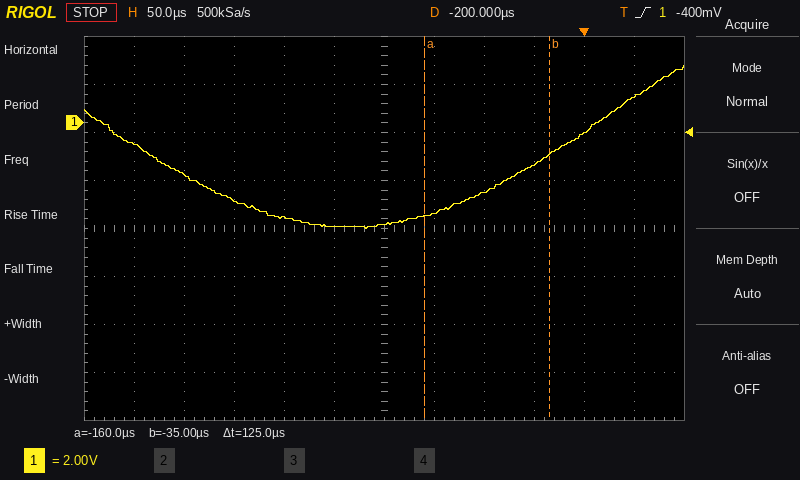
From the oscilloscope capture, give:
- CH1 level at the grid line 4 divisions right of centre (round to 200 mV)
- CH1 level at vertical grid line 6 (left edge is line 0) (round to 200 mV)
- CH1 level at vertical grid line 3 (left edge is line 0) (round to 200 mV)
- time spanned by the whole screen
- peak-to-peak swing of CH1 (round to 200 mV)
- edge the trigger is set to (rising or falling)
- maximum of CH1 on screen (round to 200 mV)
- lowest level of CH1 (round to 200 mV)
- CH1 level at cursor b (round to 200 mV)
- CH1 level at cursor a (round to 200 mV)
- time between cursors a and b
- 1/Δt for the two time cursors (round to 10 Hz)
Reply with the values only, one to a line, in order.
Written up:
-400 mV
-4.2 V
-3.2 V
600 µs
6.8 V
rising
2.4 V
-4.4 V
-1.4 V
-3.8 V
125 µs
8.00 kHz
